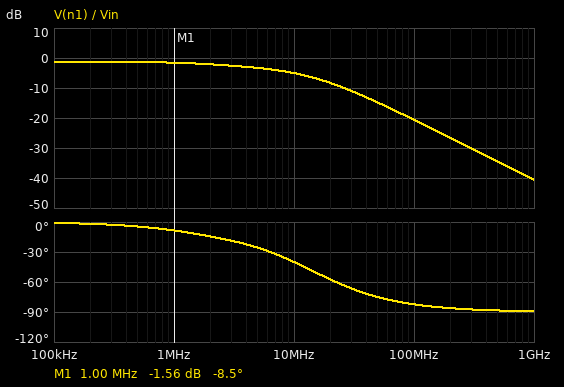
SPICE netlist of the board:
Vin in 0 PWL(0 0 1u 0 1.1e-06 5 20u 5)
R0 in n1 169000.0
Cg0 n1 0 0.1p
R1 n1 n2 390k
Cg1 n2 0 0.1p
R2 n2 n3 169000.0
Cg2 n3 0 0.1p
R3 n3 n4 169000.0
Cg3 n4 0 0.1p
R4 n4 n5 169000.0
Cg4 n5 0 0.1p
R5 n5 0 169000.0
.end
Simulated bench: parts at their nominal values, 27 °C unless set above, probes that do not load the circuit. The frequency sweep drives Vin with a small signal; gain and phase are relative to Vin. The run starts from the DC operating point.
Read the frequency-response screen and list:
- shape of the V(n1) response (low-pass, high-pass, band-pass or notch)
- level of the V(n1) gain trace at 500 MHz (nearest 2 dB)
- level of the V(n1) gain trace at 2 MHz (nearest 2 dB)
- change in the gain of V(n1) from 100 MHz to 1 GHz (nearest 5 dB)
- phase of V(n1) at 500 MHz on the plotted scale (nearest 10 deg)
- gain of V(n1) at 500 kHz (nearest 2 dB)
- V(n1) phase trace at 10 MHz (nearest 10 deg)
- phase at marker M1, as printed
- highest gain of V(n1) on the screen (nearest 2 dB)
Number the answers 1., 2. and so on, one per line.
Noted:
1. low-pass
2. -34 dB
3. -2 dB
4. -20 dB
5. -90 deg
6. -2 dB
7. -40 deg
8. -8.5 deg
9. -2 dB
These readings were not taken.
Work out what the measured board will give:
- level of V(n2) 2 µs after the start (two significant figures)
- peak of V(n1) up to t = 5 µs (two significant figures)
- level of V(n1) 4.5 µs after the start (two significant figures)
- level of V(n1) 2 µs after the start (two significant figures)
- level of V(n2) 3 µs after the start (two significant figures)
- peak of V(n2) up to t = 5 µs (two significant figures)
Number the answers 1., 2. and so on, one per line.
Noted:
1. 2.7 V
2. 4.3 V
3. 4.3 V
4. 4.3 V
5. 2.7 V
6. 2.7 V
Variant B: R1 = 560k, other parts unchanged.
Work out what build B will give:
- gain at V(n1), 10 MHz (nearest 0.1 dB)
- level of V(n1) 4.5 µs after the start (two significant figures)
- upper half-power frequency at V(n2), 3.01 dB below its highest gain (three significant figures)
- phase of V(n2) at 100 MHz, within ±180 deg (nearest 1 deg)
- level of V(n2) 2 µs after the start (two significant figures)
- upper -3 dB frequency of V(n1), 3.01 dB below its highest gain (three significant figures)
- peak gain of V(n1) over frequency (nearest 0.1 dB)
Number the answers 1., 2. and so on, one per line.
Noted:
1. -4.5 dB
2. 4.4 V
3. 2.06 MHz
4. -166 deg
5. 2.4 V
6. 8.87 MHz
7. -1.1 dB
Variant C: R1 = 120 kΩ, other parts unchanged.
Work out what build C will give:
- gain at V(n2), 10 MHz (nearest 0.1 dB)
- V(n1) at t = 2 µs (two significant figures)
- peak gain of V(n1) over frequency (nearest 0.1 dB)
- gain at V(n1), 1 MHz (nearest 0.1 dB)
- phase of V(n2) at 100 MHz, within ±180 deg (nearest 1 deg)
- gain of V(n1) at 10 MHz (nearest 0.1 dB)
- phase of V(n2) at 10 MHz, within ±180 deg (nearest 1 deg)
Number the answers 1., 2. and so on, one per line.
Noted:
1. -12.1 dB
2. 4.1 V
3. -1.7 dB
4. -2.0 dB
5. -155 deg
6. -7.2 dB
7. -75 deg
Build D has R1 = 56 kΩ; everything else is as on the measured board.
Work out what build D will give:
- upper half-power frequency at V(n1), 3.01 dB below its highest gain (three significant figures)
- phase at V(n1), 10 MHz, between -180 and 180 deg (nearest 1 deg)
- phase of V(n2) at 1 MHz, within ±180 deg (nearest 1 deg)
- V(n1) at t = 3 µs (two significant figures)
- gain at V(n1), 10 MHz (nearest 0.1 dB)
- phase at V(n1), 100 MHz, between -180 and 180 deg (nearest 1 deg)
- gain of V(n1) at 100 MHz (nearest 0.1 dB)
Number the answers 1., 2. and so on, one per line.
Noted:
1. 4.02 MHz
2. -46 deg
3. -16 deg
4. 4.1 V
5. -8.4 dB
6. -72 deg
7. -21.6 dB
